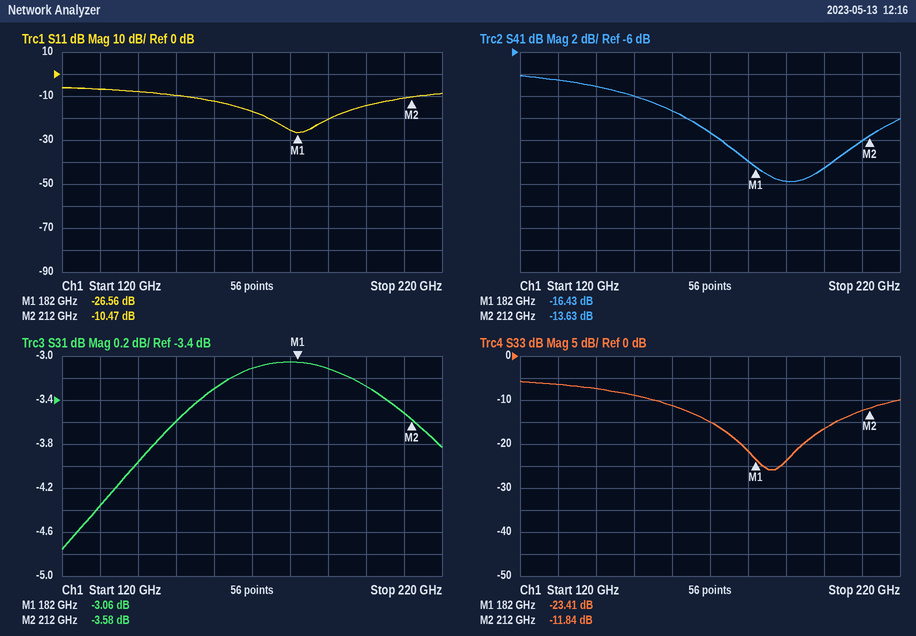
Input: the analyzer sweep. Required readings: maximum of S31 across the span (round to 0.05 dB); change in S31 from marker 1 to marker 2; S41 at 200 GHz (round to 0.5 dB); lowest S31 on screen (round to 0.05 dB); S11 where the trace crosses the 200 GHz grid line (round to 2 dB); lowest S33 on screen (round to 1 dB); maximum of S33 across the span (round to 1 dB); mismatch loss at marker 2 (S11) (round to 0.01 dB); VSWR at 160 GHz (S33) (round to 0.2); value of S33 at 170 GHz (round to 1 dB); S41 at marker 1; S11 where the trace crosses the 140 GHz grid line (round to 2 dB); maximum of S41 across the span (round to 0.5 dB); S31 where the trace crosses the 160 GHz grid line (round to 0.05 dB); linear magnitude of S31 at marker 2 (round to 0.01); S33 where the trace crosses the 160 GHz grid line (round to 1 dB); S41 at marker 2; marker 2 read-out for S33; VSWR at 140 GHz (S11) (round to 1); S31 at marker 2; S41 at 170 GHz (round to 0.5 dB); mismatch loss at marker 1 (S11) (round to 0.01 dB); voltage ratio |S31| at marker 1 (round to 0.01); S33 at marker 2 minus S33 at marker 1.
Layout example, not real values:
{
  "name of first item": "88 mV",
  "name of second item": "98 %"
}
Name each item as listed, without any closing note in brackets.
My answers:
{
  "maximum of S31 across the span": "-3.05 dB",
  "change in S31 from marker 1 to marker 2": "-0.52 dB",
  "S41 at 200 GHz": "-16.5 dB",
  "lowest S31 on screen": "-4.75 dB",
  "S11 where the trace crosses the 200 GHz grid line": "-14 dB",
  "lowest S33 on screen": "-26 dB",
  "maximum of S33 across the span": "-6 dB",
  "mismatch loss at marker 2 (S11)": "0.41 dB",
  "VSWR at 160 GHz (S33)": "1.8",
  "value of S33 at 170 GHz": "-15 dB",
  "S41 at marker 1": "-16.43 dB",
  "S11 where the trace crosses the 140 GHz grid line": "-8 dB",
  "maximum of S41 across the span": "-8.0 dB",
  "S31 where the trace crosses the 160 GHz grid line": "-3.30 dB",
  "linear magnitude of S31 at marker 2": "0.66",
  "S33 where the trace crosses the 160 GHz grid line": "-11 dB",
  "S41 at marker 2": "-13.63 dB",
  "marker 2 read-out for S33": "-11.84 dB",
  "VSWR at 140 GHz (S11)": "2",
  "S31 at marker 2": "-3.58 dB",
  "S41 at 170 GHz": "-13.5 dB",
  "mismatch loss at marker 1 (S11)": "0.01 dB",
  "voltage ratio |S31| at marker 1": "0.70",
  "S33 at marker 2 minus S33 at marker 1": "11.57 dB"
}
